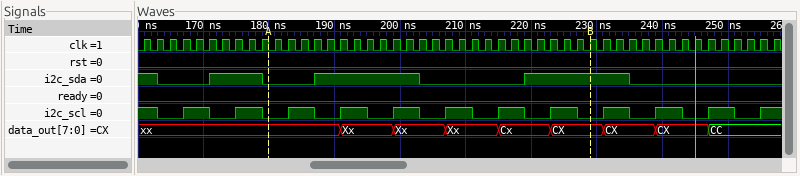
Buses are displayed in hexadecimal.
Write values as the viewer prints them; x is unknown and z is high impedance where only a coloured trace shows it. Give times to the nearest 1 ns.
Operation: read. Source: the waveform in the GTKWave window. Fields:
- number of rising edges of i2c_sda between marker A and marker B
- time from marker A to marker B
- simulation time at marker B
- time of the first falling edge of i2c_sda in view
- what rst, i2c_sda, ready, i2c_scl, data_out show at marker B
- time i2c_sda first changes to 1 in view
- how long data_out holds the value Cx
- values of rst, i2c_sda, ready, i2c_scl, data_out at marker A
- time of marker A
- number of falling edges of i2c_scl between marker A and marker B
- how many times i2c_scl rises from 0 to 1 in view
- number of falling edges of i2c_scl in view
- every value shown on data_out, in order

2
49 ns
229 ns
163 ns
rst=0, i2c_sda=1, ready=0, i2c_scl=0, data_out=CX
171 ns
8 ns
rst=0, i2c_sda=0, ready=0, i2c_scl=0, data_out=xx
180 ns
6
12
12
xx, Xx, Xx, Xx, Cx, CX, CX, CX, CC
